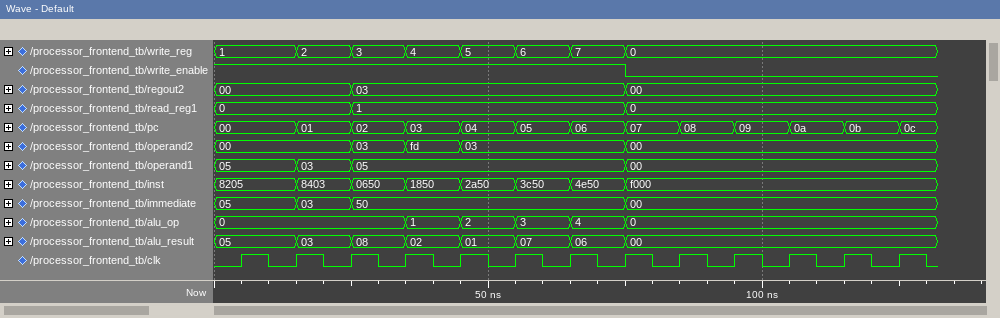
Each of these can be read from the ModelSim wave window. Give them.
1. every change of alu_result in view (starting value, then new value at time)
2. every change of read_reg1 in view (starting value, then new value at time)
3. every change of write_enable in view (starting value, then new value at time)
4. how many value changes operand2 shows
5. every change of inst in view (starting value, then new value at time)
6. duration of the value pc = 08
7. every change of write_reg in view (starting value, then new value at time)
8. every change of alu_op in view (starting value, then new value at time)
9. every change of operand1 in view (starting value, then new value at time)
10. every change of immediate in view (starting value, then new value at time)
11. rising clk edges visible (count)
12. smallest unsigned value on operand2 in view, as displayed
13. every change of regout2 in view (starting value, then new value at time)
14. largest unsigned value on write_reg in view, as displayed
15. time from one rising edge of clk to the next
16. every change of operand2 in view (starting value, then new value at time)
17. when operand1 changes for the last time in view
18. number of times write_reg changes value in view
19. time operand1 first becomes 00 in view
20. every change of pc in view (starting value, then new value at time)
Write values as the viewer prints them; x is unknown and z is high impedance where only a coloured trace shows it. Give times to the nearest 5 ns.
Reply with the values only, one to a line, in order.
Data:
05, 03 at 15 ns, 08 at 25 ns, 02 at 35 ns, 01 at 45 ns, 07 at 55 ns, 06 at 65 ns, 00 at 75 ns
0, 1 at 25 ns, 0 at 75 ns
1, 0 at 75 ns
4
8205, 8403 at 15 ns, 0650 at 25 ns, 1850 at 35 ns, 2a50 at 45 ns, 3c50 at 55 ns, 4e50 at 65 ns, f000 at 75 ns
10 ns
1, 2 at 15 ns, 3 at 25 ns, 4 at 35 ns, 5 at 45 ns, 6 at 55 ns, 7 at 65 ns, 0 at 75 ns
0, 1 at 35 ns, 2 at 45 ns, 3 at 55 ns, 4 at 65 ns, 0 at 75 ns
05, 03 at 15 ns, 05 at 25 ns, 00 at 75 ns
05, 03 at 15 ns, 50 at 25 ns, 00 at 75 ns
13
00
00, 03 at 25 ns, 00 at 75 ns
7
10 ns
00, 03 at 25 ns, fd at 35 ns, 03 at 45 ns, 00 at 75 ns
75 ns
7
75 ns
00, 01 at 15 ns, 02 at 25 ns, 03 at 35 ns, 04 at 45 ns, 05 at 55 ns, 06 at 65 ns, 07 at 75 ns, 08 at 85 ns, 09 at 95 ns, 0a at 105 ns, 0b at 115 ns, 0c at 125 ns
